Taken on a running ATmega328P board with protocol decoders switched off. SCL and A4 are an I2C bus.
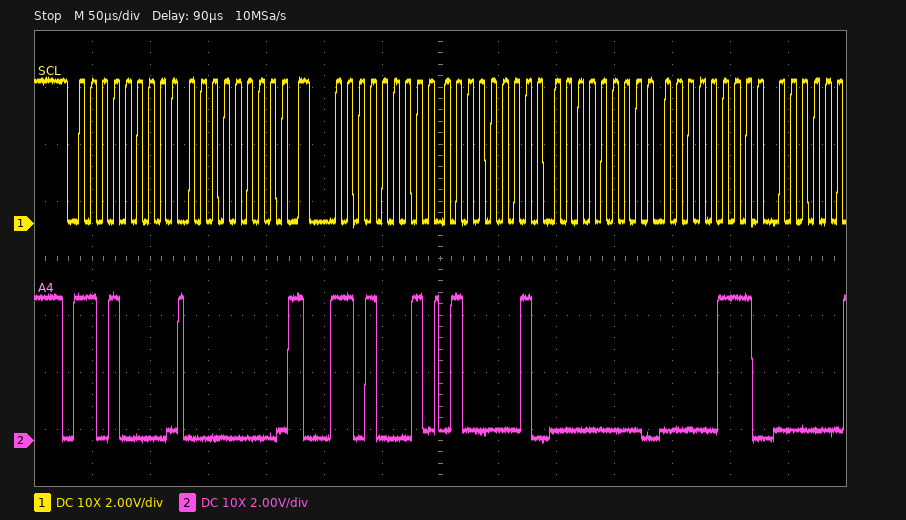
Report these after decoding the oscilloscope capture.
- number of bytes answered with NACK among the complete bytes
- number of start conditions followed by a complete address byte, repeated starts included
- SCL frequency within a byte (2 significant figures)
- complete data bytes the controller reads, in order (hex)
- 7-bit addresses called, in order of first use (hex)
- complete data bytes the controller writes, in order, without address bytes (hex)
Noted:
0
2
100 kHz
41 00 07
0x68
00
